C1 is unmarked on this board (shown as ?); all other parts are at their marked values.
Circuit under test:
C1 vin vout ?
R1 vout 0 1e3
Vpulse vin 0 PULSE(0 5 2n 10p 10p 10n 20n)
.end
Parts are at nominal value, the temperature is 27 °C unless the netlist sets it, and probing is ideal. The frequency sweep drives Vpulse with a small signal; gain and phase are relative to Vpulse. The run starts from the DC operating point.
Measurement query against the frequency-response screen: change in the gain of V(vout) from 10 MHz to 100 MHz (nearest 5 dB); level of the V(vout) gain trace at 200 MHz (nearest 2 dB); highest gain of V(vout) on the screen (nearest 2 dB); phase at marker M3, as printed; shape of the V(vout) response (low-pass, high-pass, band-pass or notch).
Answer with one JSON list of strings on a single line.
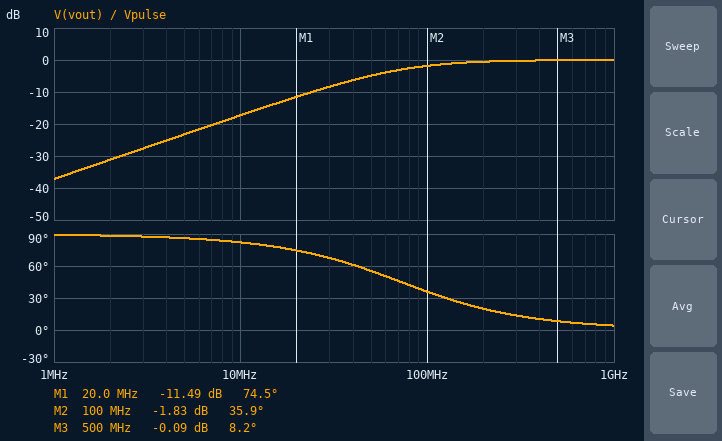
["15 dB", "0 dB", "0 dB", "8.2 deg", "high-pass"]
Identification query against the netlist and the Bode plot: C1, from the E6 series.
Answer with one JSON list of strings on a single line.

["2.2 pF"]
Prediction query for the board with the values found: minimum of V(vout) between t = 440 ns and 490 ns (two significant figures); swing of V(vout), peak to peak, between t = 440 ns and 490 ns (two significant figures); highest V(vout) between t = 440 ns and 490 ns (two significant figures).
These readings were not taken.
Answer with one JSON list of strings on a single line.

["-4.9 V", "9.9 V", "4.9 V"]
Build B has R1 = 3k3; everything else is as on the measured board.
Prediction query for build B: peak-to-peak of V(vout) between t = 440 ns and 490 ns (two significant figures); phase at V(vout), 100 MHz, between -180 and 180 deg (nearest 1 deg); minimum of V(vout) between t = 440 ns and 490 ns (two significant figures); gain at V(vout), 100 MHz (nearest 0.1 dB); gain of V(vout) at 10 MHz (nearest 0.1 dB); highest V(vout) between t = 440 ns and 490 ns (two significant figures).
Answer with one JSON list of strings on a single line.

["8.0 V", "12 deg", "-4.0 V", "-0.2 dB", "-7.6 dB", "4.0 V"]
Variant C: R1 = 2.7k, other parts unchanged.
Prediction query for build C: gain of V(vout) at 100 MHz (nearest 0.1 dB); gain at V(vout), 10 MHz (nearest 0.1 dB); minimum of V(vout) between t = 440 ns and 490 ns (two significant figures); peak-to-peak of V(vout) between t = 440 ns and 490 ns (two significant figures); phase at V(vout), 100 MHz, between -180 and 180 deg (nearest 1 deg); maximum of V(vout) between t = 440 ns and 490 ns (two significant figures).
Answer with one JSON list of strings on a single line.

["-0.3 dB", "-9.1 dB", "-4.2 V", "8.4 V", "15 deg", "4.2 V"]
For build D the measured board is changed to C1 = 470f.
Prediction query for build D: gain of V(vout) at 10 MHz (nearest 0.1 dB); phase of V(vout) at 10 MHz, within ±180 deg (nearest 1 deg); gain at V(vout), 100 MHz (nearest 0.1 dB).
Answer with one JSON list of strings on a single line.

["-30.6 dB", "88 deg", "-11.0 dB"]
